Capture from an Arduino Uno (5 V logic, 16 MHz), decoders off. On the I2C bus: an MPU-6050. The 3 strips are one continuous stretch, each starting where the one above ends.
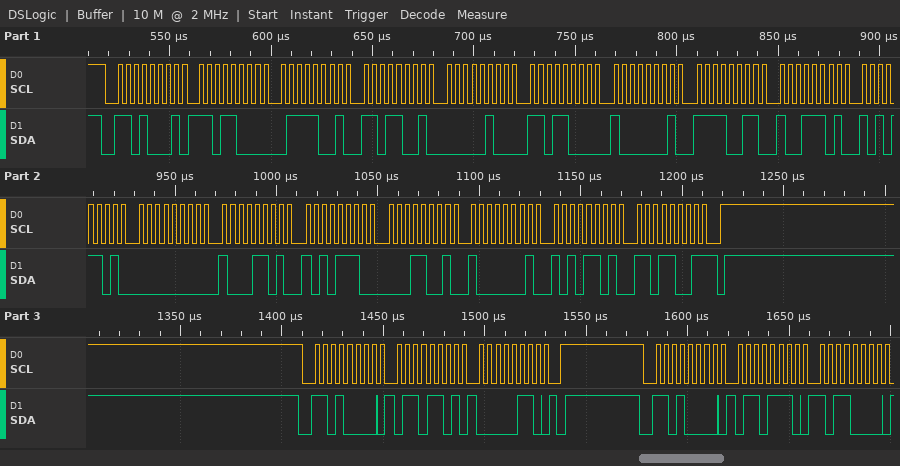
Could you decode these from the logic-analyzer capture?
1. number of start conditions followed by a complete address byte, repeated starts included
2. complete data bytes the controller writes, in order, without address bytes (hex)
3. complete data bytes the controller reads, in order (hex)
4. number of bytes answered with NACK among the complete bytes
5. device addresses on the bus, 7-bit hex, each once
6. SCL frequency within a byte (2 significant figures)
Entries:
3
6D 06 6E B0
D8 79 D9 04 D8 81 F3 9D AD 00 8D AE 19 81 AD D9
1
0x68
250 kHz
